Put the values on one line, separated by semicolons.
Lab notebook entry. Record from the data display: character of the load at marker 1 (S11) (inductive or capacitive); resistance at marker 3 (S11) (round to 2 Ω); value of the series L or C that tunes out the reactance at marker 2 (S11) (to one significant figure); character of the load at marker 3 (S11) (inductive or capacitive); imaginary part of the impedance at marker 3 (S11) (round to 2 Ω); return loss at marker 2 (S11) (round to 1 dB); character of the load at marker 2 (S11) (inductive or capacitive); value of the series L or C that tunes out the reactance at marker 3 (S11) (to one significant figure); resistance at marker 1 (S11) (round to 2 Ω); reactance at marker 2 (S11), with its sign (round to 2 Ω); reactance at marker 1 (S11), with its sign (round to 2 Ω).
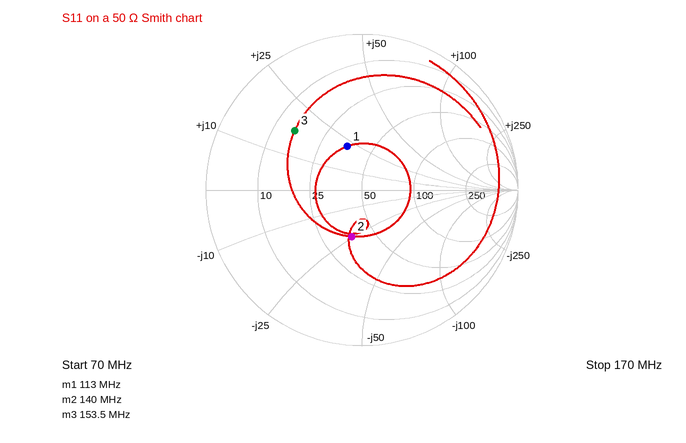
inductive; 16 Ω; 30 nH; inductive; +18 Ω; 10 dB; capacitive; 60 pF; 36 Ω; -24 Ω; +22 Ω
